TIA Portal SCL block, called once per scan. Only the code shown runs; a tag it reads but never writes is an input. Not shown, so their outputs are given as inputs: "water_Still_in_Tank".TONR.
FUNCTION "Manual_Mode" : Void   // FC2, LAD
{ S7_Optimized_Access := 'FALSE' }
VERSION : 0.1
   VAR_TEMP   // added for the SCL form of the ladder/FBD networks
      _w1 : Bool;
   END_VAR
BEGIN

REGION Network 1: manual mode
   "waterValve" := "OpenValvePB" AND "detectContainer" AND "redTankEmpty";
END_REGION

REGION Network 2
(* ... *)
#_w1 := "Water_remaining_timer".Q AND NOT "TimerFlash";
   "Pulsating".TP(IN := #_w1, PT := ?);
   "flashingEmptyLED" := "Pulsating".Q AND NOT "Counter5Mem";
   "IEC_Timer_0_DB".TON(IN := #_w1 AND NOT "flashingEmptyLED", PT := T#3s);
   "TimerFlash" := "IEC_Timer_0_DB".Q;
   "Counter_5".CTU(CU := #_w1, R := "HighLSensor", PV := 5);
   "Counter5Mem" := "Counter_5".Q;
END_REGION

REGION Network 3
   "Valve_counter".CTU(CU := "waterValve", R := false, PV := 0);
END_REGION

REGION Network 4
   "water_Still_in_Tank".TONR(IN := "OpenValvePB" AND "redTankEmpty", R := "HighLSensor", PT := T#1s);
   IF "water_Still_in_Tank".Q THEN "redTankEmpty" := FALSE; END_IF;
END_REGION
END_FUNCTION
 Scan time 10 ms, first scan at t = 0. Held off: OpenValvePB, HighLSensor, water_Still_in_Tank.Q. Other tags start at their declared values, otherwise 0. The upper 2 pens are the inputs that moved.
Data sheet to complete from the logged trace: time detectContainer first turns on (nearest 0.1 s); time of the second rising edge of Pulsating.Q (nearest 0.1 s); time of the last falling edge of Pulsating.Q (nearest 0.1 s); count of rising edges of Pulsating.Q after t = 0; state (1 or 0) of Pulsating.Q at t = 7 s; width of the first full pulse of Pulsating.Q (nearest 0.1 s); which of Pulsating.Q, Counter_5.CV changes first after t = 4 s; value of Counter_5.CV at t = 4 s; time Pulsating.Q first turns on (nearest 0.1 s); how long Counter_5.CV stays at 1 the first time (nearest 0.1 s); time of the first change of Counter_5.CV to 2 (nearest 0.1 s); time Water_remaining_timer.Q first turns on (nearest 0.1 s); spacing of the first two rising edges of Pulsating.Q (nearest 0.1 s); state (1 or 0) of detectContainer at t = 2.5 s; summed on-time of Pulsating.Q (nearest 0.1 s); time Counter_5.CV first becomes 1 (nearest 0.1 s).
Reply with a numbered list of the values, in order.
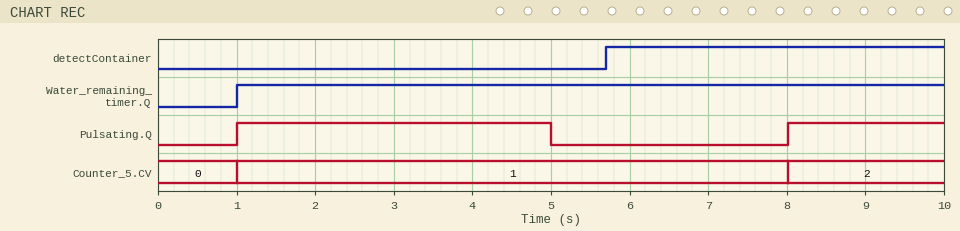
1. 5.7 s
2. 8.0 s
3. 5.0 s
4. 2
5. 0
6. 4.0 s
7. Pulsating.Q
8. 1
9. 1.0 s
10. 7.0 s
11. 8.0 s
12. 1.0 s
13. 7.0 s
14. 0
15. 6.0 s
16. 1.0 s
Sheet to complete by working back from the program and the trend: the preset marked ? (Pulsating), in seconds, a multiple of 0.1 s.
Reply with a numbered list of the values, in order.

1. 4.0 s
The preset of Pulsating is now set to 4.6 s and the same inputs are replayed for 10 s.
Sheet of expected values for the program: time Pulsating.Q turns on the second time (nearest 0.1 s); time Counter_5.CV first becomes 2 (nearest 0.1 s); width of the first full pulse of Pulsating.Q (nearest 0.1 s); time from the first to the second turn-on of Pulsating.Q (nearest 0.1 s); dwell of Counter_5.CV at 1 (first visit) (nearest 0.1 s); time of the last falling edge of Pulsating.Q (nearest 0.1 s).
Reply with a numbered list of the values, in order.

1. 8.6 s
2. 8.6 s
3. 4.6 s
4. 7.6 s
5. 7.6 s
6. 5.6 s
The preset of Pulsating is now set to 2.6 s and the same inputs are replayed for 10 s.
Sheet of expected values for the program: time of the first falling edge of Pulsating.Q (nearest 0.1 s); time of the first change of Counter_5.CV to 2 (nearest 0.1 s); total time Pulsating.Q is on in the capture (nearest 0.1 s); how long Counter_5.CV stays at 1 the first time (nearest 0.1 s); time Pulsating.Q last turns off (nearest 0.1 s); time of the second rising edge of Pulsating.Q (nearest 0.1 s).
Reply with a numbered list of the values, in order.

1. 3.6 s
2. 6.6 s
3. 5.2 s
4. 5.6 s
5. 9.2 s
6. 6.6 s
